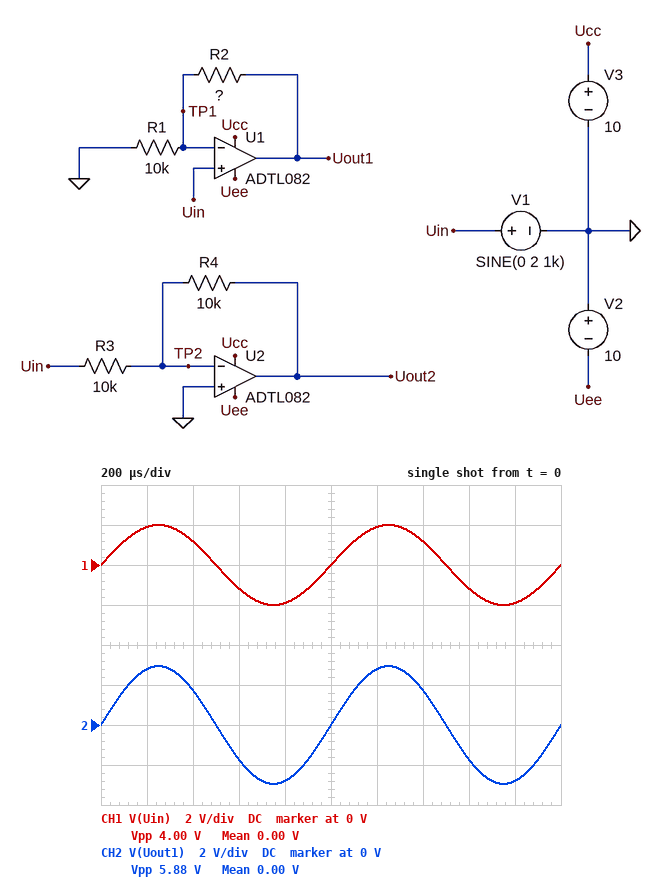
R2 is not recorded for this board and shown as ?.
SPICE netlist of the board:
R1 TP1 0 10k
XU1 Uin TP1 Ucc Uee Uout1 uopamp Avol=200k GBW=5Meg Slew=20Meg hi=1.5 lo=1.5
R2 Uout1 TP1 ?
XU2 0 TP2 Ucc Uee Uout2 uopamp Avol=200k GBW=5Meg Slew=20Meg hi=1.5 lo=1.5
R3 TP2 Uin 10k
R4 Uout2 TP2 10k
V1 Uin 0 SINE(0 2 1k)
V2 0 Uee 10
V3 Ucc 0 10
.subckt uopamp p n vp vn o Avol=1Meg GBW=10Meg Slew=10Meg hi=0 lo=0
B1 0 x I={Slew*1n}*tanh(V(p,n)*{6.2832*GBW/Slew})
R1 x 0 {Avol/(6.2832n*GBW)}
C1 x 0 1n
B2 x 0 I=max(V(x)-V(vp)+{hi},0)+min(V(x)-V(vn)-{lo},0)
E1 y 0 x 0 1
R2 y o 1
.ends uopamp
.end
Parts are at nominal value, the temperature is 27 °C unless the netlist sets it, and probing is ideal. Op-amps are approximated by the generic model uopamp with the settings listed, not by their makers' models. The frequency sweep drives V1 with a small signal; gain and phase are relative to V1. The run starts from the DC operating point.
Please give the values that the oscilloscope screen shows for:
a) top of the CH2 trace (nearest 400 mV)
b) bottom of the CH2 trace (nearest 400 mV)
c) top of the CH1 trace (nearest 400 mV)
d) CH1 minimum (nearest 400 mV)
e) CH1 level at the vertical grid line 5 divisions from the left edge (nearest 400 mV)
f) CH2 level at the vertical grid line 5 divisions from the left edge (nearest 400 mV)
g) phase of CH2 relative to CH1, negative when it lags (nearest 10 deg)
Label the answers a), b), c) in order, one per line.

a) 2.8 V
b) -2.8 V
c) 2.0 V
d) -2.0 V
e) 0 V
f) 0 V
g) 0 deg
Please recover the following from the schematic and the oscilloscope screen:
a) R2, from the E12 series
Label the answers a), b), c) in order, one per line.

a) 4.7 kΩ
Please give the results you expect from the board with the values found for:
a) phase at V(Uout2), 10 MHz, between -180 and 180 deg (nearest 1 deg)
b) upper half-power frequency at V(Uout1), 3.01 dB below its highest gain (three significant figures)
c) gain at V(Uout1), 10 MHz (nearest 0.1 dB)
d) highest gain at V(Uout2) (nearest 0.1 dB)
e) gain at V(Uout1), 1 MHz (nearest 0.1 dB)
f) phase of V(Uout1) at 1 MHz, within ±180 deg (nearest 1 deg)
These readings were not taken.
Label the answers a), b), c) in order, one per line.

a) 104 deg
b) 3.40 MHz
c) -6.5 dB
d) 0 dB
e) 3.0 dB
f) -16 deg
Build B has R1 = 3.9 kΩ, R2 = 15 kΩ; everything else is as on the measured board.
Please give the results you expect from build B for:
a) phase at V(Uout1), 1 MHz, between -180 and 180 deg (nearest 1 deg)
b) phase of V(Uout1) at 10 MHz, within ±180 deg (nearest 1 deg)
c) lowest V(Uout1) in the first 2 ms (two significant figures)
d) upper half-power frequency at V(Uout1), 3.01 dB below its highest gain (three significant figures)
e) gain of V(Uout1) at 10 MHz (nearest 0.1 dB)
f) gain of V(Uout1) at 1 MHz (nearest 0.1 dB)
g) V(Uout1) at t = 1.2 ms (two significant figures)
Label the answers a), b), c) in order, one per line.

a) -44 deg
b) -84 deg
c) -8.5 V
d) 1.03 MHz
e) -6.1 dB
f) 10.8 dB
g) 8.5 V
